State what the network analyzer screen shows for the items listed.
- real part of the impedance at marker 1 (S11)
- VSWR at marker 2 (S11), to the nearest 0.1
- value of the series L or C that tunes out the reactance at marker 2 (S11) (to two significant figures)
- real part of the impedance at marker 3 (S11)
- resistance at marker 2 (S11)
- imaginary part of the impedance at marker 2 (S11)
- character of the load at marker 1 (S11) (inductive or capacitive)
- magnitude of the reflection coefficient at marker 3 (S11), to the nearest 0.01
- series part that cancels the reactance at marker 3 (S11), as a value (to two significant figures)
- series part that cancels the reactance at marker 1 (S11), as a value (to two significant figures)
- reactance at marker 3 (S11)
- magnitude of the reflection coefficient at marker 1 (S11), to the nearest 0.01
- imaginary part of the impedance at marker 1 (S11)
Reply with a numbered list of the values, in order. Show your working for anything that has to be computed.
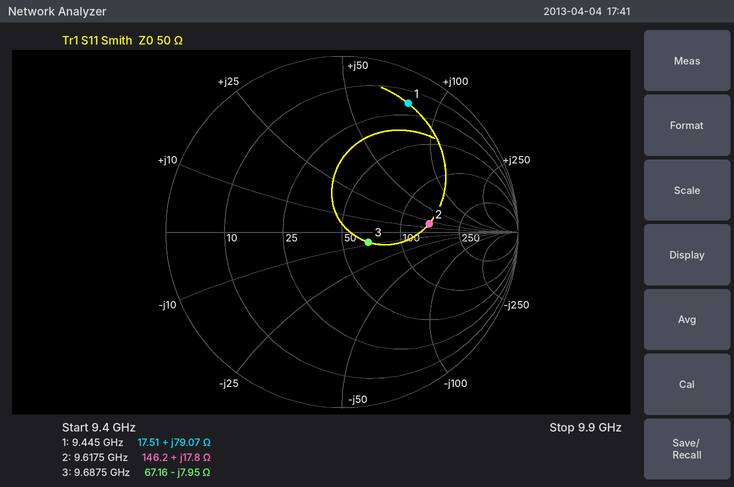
1. 17.51 Ω
2. 3.0
3. C = 1/(2π × 9.6175 GHz × 17.8 Ω) ≈ 930 fF
4. 67.16 Ω
5. 146.2 Ω
6. +17.8 Ω
7. inductive
8. 0.16
9. L = 7.95 Ω/(2π × 9.6875 GHz) ≈ 131 pH, so 130 pH to two significant figures
10. C = 1/(2π × 9.445 GHz × 79.07 Ω) ≈ 213 fF, so 210 fF to two significant figures
11. -7.95 Ω
12. 0.82
13. +79.07 Ω
